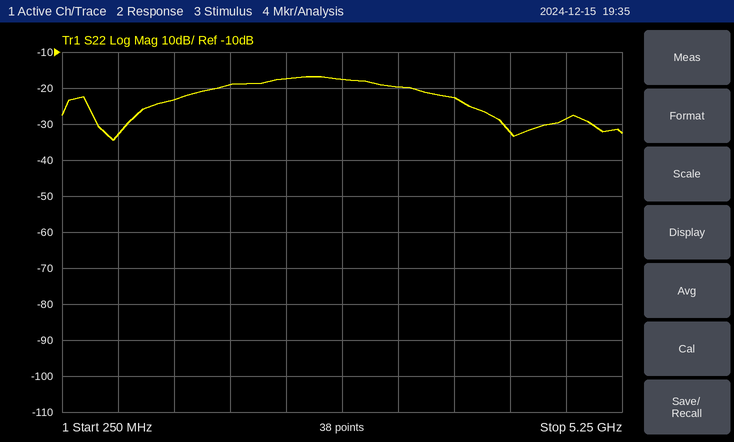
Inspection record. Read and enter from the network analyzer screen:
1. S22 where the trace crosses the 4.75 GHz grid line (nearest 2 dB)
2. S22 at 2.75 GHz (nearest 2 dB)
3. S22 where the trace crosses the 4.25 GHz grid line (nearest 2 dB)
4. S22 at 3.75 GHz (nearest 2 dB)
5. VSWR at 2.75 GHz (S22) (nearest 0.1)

-28 dB
-18 dB
-32 dB
-22 dB
1.3
